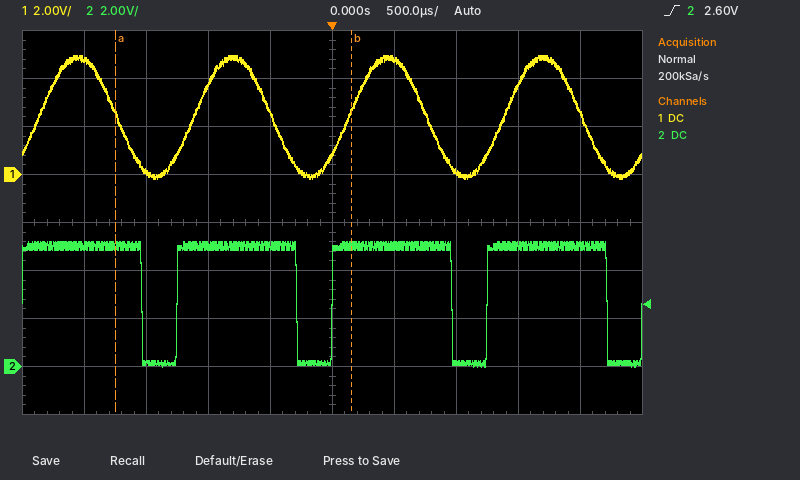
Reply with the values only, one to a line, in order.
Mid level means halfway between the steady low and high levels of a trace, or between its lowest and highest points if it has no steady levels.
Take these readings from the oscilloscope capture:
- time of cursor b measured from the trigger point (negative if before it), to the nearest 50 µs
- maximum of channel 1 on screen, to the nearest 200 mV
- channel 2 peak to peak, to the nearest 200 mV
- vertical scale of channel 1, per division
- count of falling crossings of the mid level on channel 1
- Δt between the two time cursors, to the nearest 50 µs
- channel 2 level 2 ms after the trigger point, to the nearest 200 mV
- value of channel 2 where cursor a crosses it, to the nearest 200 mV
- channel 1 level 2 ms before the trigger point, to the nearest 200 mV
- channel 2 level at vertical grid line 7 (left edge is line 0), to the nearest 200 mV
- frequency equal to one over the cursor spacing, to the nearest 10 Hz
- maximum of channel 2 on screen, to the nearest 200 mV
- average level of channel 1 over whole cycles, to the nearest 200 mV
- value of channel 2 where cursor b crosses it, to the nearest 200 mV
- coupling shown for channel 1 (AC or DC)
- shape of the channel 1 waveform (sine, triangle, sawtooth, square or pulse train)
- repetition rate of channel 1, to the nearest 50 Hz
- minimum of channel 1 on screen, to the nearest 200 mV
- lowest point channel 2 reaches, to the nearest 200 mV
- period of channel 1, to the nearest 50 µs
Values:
+150 µs
5.0 V
5.2 V
2 V
4
1.90 ms
5.0 V
5.0 V
4.8 V
200 mV
530 Hz
5.2 V
2.4 V
5.0 V
DC
sine
800 Hz
-200 mV
0.0 V
1.25 ms
